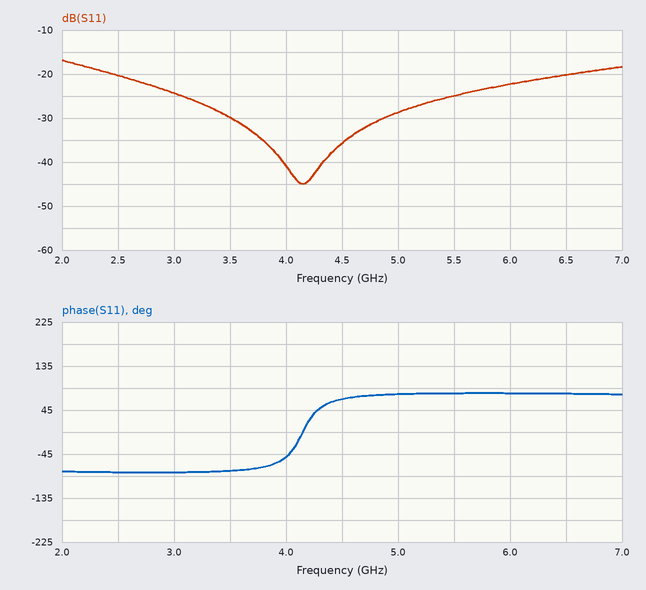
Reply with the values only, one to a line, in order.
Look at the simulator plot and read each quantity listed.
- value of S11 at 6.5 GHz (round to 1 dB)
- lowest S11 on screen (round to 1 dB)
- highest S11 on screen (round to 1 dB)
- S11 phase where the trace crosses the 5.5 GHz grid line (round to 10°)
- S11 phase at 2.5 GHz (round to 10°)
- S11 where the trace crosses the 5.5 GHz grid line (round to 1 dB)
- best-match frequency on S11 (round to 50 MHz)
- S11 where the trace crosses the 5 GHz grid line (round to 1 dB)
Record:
-20 dB
-45 dB
-17 dB
80°
-80°
-25 dB
4.15 GHz
-29 dB
